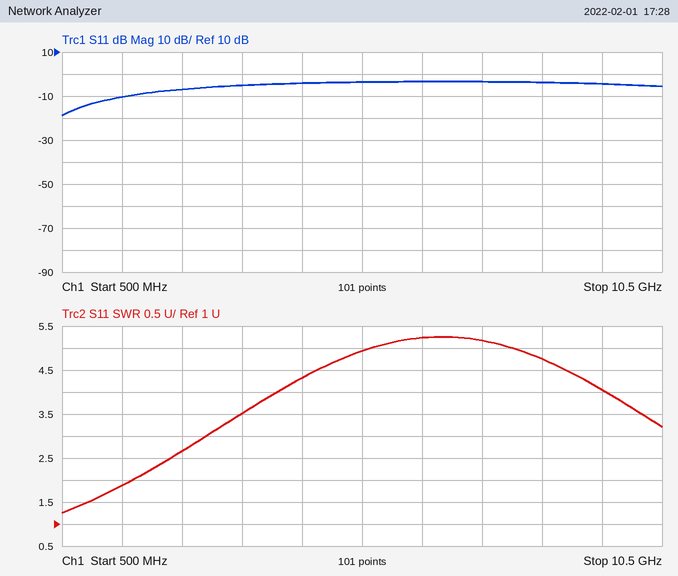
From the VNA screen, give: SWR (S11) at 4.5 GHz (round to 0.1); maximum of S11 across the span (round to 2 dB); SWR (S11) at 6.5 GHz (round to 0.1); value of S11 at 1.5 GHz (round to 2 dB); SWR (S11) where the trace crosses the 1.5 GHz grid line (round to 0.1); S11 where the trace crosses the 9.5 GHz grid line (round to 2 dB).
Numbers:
4.3
-4 dB
5.2
-10 dB
1.9
-4 dB
